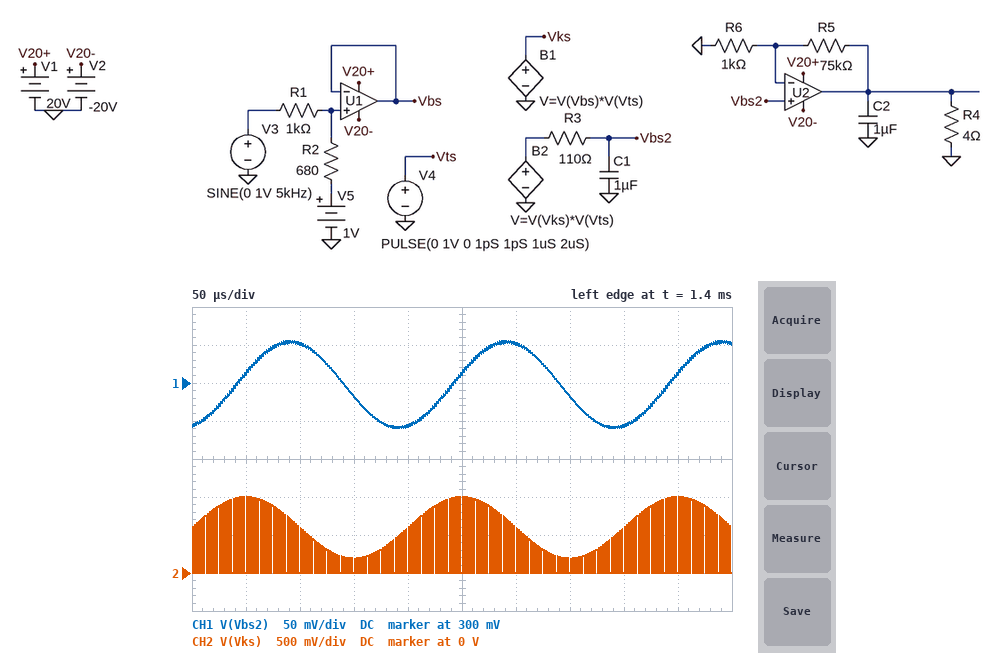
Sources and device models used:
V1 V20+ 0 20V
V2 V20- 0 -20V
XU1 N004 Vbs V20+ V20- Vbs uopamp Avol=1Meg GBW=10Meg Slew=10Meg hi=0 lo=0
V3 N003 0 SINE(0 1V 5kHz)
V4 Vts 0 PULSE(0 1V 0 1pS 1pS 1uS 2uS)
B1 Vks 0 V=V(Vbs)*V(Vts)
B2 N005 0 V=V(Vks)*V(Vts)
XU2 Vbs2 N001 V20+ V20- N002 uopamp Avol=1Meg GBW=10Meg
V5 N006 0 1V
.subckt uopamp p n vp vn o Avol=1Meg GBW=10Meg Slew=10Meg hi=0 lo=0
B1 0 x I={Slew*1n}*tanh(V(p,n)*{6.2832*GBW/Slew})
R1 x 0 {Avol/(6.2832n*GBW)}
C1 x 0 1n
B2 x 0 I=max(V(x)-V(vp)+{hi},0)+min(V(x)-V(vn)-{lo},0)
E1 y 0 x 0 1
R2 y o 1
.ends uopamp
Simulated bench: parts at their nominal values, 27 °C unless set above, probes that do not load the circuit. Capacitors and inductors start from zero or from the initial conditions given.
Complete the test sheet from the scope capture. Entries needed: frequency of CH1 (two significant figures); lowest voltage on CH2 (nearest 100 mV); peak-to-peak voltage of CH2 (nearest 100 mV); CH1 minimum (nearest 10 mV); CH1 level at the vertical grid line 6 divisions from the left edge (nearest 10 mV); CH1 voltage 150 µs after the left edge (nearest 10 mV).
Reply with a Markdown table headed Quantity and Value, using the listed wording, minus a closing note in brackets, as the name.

| Quantity | Value |
|---|---|
| frequency of CH1 | 5.0 kHz |
| lowest voltage on CH2 | 0 V |
| peak-to-peak voltage of CH2 | 1.0 V |
| CH1 minimum | 240 mV |
| CH1 level at the vertical grid line 6 divisions from the left edge | 350 mV |
| CH1 voltage 150 µs after the left edge | 280 mV |
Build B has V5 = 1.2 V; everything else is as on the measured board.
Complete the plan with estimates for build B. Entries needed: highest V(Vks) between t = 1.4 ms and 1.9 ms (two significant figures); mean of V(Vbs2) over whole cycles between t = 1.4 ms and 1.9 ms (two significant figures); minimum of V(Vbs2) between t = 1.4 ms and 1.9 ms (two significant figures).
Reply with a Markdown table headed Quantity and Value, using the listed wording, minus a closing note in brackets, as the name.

| Quantity | Value |
|---|---|
| highest V(Vks) between t = 1.4 ms and 1.9 ms | 1.1 V |
| mean of V(Vbs2) over whole cycles between t = 1.4 ms and 1.9 ms | 360 mV |
| minimum of V(Vbs2) between t = 1.4 ms and 1.9 ms | 300 mV |
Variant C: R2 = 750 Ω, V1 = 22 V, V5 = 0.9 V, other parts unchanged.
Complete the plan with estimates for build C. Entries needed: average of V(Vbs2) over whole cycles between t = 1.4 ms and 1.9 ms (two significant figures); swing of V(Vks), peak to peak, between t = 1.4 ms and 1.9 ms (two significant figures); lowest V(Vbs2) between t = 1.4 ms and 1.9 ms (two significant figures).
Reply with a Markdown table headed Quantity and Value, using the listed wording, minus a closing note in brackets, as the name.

| Quantity | Value |
|---|---|
| average of V(Vbs2) over whole cycles between t = 1.4 ms and 1.9 ms | 260 mV |
| swing of V(Vks), peak to peak, between t = 1.4 ms and 1.9 ms | 940 mV |
| lowest V(Vbs2) between t = 1.4 ms and 1.9 ms | 200 mV |
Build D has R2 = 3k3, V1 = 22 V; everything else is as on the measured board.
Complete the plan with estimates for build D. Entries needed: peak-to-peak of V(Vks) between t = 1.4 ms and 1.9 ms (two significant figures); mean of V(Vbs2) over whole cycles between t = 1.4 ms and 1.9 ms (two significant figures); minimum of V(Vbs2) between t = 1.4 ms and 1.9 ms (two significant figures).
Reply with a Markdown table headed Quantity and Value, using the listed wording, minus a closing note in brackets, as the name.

| Quantity | Value |
|---|---|
| peak-to-peak of V(Vks) between t = 1.4 ms and 1.9 ms | 1.5 V |
| mean of V(Vbs2) over whole cycles between t = 1.4 ms and 1.9 ms | 120 mV |
| minimum of V(Vbs2) between t = 1.4 ms and 1.9 ms | 9.6 mV |
